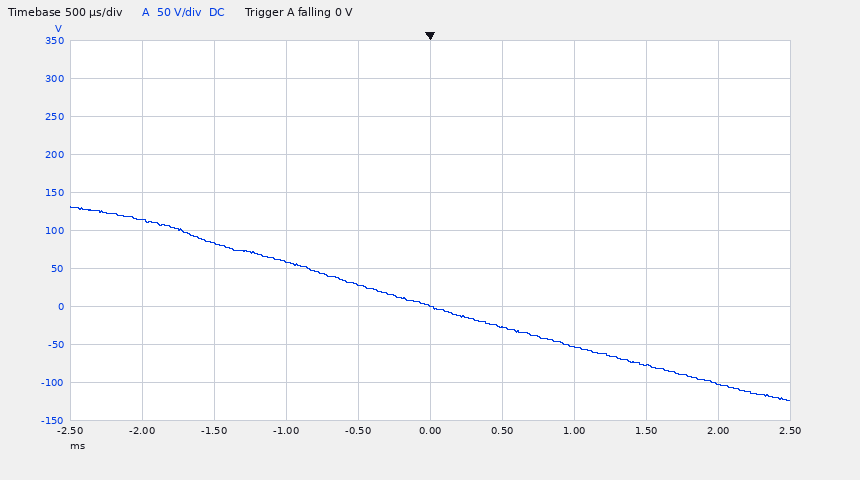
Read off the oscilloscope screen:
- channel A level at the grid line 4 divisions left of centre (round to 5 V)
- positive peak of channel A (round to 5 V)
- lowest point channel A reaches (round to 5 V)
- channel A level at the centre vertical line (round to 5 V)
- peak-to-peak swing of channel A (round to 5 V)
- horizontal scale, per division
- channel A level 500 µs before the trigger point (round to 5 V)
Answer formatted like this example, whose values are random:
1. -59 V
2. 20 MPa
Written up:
1. 115 V
2. 130 V
3. -125 V
4. 0 V
5. 255 V
6. 500 µs
7. 30 V
